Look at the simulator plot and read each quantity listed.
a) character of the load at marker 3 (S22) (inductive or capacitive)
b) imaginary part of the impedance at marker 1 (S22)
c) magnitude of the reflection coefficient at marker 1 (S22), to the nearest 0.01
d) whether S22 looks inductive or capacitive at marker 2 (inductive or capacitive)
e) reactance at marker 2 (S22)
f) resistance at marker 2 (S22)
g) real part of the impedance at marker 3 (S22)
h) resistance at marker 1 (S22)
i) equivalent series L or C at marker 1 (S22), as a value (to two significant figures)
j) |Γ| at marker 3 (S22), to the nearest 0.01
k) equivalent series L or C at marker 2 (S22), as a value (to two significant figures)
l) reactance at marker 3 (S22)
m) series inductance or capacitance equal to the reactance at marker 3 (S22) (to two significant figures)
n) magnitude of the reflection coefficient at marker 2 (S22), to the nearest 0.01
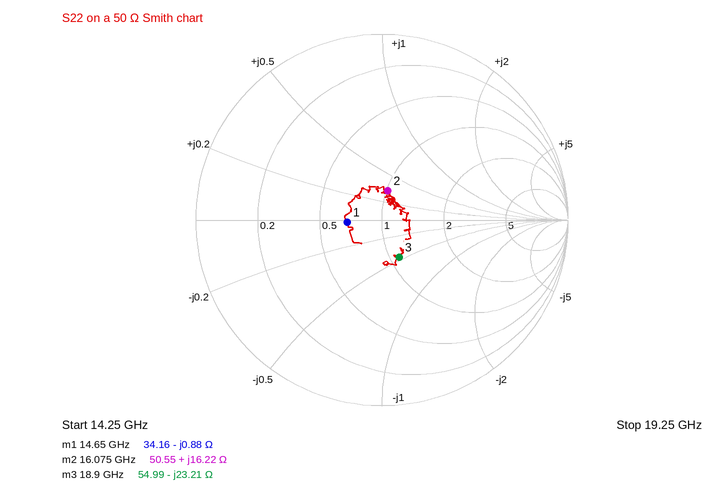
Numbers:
capacitive
-0.88 Ω
0.19
inductive
+16.22 Ω
50.55 Ω
54.99 Ω
34.16 Ω
12 pF
0.22
160 pH
-23.21 Ω
360 fF
0.16
